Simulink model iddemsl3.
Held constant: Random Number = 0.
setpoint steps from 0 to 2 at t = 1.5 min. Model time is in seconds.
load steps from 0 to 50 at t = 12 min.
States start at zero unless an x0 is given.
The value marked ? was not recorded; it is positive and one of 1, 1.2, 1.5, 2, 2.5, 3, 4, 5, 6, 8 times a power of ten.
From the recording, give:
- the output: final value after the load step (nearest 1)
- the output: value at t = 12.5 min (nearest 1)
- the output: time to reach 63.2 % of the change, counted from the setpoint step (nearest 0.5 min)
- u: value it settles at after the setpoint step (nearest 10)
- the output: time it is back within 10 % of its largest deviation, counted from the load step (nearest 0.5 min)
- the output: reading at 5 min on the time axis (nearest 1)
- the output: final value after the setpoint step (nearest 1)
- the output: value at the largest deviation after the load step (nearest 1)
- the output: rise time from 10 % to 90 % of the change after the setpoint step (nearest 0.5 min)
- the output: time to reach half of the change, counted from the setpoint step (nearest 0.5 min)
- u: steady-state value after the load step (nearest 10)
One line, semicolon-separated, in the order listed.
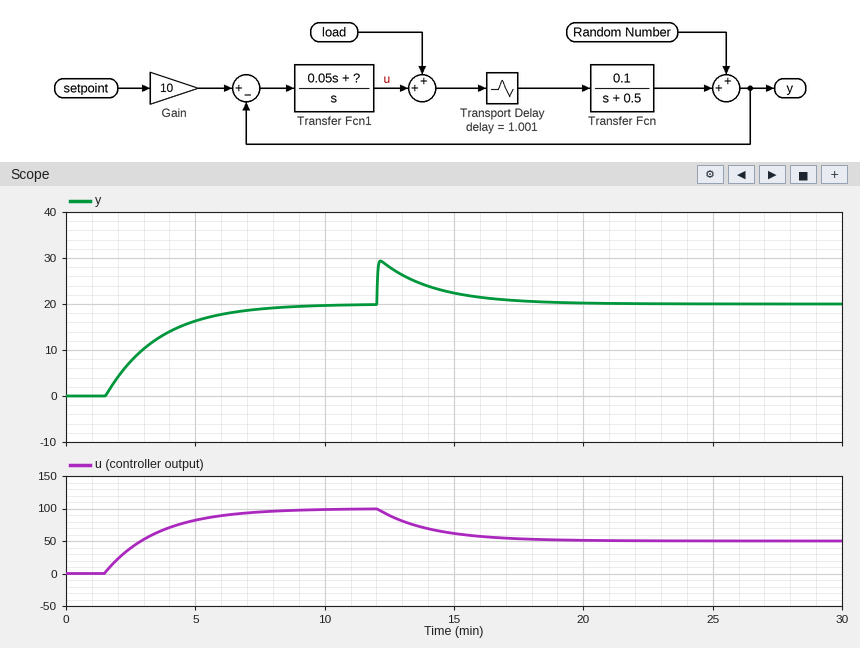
20; 28; 2.0 min; 100; 5.0 min; 16; 20; 29; 4.5 min; 1.5 min; 50
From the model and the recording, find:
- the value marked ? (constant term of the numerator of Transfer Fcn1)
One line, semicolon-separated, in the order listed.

0.04
